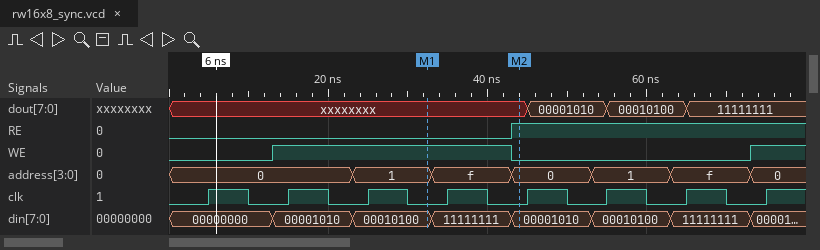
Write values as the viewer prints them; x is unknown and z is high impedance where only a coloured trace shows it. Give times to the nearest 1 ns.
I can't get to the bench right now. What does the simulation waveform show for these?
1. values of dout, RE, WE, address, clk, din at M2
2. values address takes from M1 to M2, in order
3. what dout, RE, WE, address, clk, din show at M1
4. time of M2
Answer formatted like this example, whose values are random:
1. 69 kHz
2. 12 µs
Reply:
1. dout=xxxxxxxx, RE=1, WE=0, address=0, clk=0, din=00001010
2. 1, f, 0
3. dout=xxxxxxxx, RE=0, WE=1, address=1, clk=0, din=00010100
4. 44 ns
